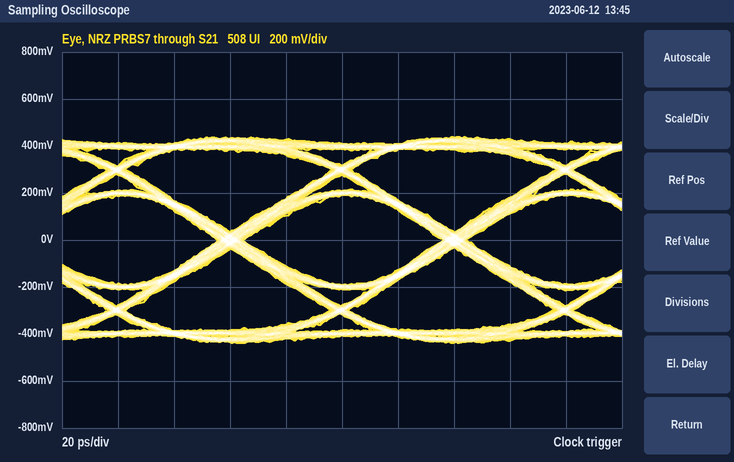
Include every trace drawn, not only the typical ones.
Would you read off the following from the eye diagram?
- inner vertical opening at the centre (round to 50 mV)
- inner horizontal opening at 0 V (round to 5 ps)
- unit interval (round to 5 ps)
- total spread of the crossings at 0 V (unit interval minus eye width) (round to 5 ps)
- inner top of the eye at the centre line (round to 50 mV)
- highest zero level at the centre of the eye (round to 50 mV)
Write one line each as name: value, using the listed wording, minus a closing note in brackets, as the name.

inner vertical opening at the centre: 400 mV
inner horizontal opening at 0 V: 70 ps
unit interval: 80 ps
total spread of the crossings at 0 V (unit interval minus eye width): 10 ps
inner top of the eye at the centre line: 200 mV
highest zero level at the centre of the eye: -200 mV
